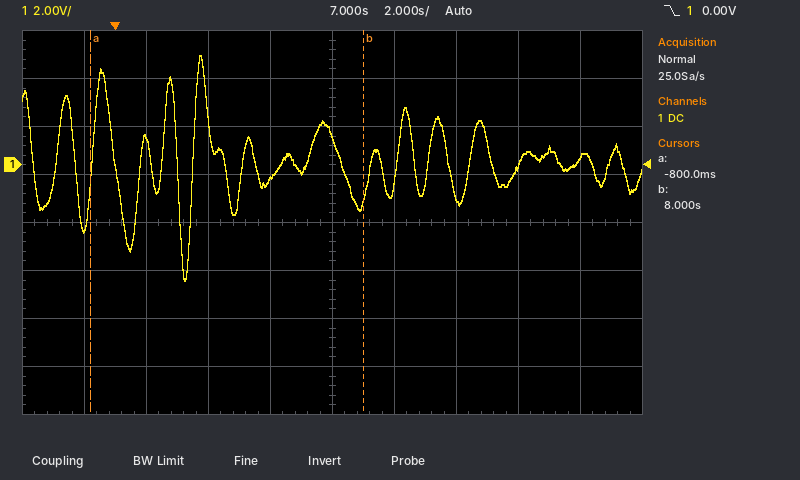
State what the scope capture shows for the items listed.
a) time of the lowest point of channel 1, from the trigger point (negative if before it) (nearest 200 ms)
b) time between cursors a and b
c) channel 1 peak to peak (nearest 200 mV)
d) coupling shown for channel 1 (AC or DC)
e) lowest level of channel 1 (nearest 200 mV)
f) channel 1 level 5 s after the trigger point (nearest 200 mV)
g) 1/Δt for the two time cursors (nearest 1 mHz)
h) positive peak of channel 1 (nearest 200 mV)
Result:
+2.2 s
8.8 s
9.4 V
DC
-4.8 V
-600 mV
114 mHz
4.6 V
